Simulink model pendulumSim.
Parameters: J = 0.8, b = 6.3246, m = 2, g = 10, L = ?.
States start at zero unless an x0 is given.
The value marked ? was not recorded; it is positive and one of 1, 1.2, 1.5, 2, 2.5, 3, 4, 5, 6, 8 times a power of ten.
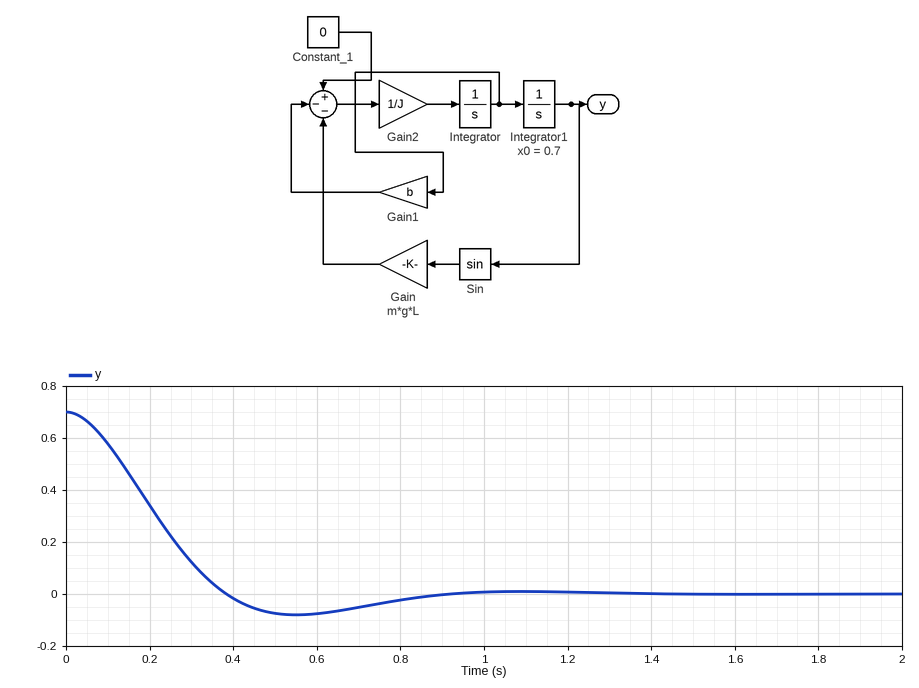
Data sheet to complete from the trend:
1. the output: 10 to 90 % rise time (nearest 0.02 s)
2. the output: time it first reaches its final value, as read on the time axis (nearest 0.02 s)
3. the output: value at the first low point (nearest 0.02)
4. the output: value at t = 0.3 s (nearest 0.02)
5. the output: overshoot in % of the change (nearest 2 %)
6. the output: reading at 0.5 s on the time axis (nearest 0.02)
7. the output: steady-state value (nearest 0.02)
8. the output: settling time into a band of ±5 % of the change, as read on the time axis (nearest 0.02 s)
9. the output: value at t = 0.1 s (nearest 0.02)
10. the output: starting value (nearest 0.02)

0.26 s
0.38 s
-0.08
0.12
12 %
-0.08
0.00
0.76 s
0.58
0.70
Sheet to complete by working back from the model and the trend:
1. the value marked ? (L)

2
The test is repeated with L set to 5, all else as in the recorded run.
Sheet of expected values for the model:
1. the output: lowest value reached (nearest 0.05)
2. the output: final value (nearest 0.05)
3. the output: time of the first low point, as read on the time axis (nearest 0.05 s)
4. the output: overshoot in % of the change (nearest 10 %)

-0.20
0.00
0.30 s
30 %
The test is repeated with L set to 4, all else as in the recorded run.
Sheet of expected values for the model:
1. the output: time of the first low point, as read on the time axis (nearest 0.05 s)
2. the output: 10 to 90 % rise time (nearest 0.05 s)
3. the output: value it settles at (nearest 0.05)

0.35 s
0.15 s
0.00
